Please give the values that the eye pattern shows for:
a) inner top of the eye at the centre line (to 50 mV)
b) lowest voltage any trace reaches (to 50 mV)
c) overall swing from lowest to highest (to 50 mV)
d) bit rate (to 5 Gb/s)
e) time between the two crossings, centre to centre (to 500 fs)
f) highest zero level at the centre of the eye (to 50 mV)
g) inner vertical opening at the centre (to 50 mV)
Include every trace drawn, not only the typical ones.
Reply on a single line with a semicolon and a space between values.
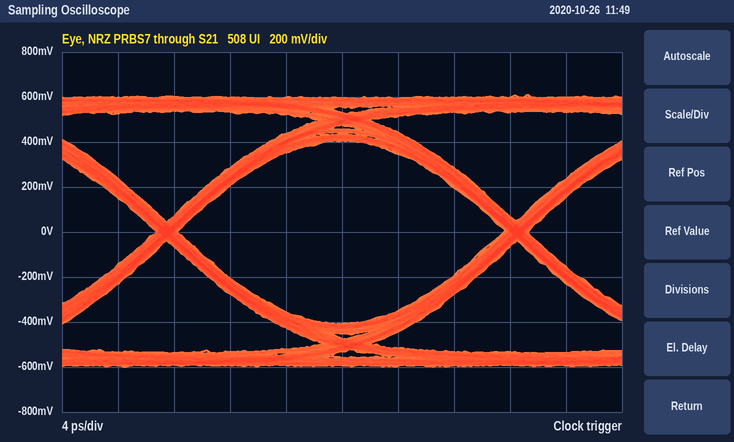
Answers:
400 mV; -600 mV; 1.20 V; 40 Gb/s; 25.0 ps; -400 mV; 800 mV
